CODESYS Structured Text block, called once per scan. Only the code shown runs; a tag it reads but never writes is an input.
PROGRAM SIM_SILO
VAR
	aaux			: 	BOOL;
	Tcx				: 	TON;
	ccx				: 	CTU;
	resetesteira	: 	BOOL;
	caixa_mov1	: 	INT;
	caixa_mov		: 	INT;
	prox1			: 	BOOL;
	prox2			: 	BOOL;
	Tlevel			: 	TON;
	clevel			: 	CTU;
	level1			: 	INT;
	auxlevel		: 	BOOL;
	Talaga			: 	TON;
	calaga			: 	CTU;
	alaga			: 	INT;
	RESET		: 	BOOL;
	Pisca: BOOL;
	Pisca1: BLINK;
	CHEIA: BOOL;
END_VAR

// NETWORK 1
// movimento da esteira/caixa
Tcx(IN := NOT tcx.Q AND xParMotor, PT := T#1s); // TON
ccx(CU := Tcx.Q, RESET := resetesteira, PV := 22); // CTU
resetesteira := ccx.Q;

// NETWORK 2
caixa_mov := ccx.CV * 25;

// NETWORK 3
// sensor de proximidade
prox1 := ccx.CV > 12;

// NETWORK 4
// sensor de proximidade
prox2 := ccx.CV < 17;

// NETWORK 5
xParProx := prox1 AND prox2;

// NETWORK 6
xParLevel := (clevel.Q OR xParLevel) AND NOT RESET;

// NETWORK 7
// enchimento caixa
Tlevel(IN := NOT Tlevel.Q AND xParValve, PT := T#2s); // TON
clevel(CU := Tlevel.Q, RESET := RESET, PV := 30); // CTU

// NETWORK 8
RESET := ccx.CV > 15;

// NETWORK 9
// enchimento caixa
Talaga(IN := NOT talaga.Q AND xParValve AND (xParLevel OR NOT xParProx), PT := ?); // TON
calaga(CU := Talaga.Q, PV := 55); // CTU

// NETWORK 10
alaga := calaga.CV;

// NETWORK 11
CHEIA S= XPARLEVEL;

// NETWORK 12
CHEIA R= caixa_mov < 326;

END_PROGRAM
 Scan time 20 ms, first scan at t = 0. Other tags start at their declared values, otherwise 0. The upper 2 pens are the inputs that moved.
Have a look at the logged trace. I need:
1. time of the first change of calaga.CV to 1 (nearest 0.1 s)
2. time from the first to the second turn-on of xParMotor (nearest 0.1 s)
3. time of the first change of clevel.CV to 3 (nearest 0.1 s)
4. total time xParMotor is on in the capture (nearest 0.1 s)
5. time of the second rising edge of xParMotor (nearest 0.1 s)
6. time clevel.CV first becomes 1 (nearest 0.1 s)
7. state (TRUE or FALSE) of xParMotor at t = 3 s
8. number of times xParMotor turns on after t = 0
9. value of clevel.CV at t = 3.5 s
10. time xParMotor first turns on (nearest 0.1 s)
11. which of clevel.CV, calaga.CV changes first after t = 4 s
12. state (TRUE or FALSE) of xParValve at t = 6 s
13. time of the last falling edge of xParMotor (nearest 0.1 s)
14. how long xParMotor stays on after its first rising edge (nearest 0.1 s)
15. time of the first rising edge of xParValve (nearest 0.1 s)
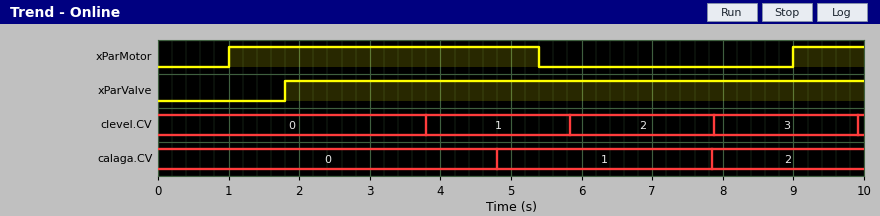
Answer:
4.8 s
8.0 s
7.9 s
5.4 s
9.0 s
3.8 s
TRUE
2
0
1.0 s
calaga.CV
TRUE
5.4 s
4.4 s
1.8 s
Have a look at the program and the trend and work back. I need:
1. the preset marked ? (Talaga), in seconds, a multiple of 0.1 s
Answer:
3.0 s
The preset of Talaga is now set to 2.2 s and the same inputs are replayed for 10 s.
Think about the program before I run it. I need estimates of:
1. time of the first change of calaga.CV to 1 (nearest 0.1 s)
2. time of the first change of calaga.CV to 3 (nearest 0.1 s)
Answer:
4.0 s
8.5 s
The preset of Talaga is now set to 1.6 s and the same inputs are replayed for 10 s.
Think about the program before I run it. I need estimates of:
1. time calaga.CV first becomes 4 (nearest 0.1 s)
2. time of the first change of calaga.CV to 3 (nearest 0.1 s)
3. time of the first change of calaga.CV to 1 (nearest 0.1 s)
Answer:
8.3 s
6.7 s
3.4 s
